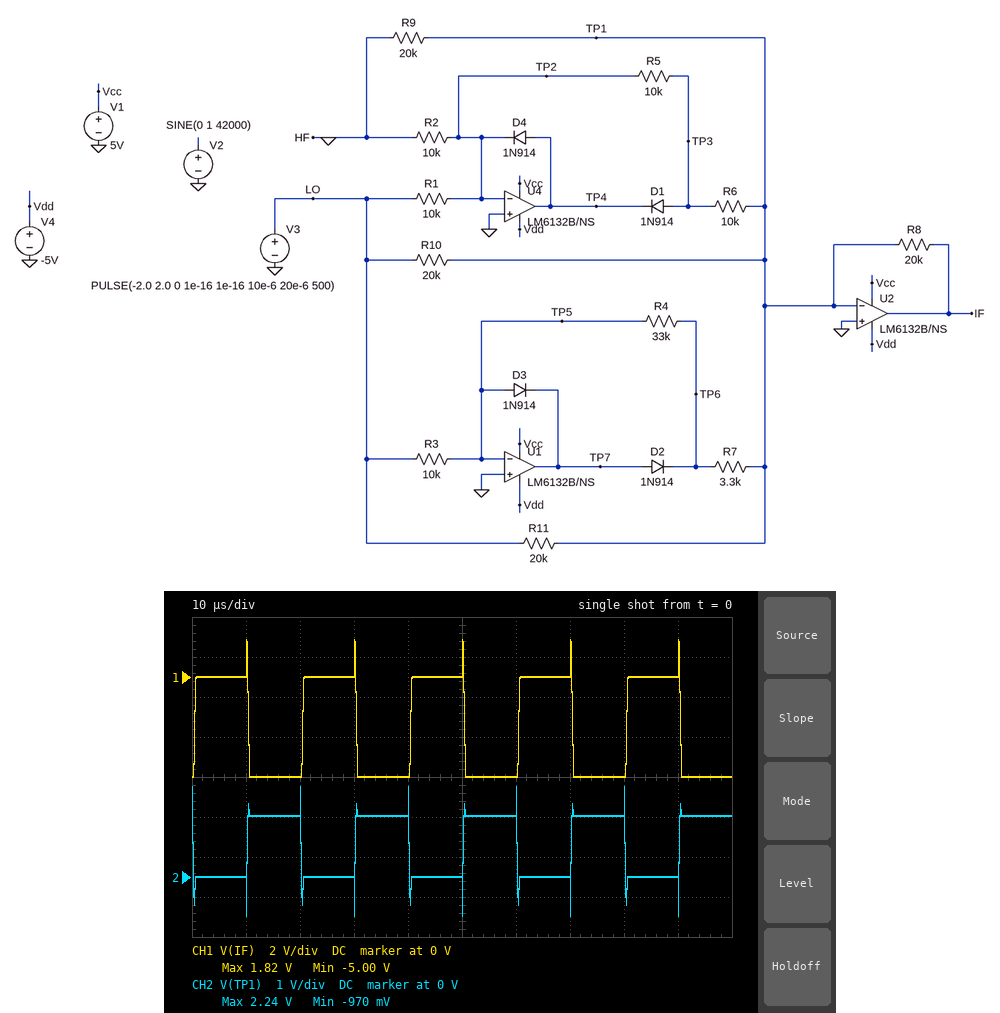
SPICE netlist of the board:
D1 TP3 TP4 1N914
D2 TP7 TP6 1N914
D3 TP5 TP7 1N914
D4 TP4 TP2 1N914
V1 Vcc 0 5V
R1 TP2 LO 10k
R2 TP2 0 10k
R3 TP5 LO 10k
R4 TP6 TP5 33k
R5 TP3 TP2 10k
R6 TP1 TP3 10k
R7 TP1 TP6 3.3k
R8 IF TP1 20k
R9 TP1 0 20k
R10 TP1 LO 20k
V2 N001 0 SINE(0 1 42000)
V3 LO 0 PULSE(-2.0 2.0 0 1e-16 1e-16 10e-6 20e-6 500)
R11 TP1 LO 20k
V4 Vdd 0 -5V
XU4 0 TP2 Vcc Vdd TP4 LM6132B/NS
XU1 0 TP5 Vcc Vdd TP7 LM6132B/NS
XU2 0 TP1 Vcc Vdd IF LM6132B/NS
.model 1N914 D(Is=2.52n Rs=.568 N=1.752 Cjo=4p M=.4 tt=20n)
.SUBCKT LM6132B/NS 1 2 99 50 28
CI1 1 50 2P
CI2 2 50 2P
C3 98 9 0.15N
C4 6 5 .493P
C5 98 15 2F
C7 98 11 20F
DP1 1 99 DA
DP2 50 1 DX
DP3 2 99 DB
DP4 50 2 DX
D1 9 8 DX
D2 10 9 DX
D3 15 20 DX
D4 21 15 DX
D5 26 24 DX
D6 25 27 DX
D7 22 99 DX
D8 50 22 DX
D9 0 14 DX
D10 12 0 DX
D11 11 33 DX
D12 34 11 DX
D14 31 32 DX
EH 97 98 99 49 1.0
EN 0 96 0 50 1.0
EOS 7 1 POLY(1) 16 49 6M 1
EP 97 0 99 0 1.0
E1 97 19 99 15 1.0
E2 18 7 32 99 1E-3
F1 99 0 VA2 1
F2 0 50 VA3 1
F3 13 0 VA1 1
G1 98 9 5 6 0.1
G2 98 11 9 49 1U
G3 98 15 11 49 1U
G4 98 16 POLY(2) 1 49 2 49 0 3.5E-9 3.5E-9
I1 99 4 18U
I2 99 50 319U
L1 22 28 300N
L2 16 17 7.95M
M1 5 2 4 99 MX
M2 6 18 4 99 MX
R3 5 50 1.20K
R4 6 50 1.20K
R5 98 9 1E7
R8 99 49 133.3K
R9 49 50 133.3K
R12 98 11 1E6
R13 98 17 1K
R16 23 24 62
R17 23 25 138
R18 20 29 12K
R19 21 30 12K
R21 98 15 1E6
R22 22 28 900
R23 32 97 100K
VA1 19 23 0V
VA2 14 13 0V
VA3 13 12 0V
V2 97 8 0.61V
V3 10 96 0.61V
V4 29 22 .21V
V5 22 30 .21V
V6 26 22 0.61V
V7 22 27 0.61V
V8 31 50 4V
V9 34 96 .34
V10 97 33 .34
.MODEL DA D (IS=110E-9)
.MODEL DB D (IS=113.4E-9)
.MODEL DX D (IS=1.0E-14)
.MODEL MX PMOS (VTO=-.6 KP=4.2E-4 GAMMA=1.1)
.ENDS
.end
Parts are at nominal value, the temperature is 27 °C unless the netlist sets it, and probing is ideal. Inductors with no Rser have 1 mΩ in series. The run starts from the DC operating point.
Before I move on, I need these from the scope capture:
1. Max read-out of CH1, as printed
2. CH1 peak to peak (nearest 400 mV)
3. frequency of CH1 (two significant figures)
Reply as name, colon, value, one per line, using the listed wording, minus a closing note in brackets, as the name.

Max read-out of CH1, as printed: 1.82 V
CH1 peak to peak: 6.8 V
frequency of CH1: 50 kHz
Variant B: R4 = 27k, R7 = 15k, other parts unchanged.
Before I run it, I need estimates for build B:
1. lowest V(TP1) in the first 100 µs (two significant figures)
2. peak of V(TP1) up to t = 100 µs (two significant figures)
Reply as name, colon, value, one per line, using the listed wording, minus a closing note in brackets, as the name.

lowest V(TP1) in the first 100 µs: -1.1 V
peak of V(TP1) up to t = 100 µs: 1.2 V
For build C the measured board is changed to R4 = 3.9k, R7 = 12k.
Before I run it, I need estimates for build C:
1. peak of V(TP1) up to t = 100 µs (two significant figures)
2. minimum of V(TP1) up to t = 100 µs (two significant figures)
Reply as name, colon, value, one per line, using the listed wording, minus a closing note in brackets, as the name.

peak of V(TP1) up to t = 100 µs: 1.1 V
minimum of V(TP1) up to t = 100 µs: -1.1 V
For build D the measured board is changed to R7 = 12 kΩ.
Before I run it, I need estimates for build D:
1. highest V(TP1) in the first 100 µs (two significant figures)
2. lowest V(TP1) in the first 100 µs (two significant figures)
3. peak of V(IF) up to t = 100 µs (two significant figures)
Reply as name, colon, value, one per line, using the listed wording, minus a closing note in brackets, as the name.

highest V(TP1) in the first 100 µs: 1.1 V
lowest V(TP1) in the first 100 µs: -1.1 V
peak of V(IF) up to t = 100 µs: 2.4 V
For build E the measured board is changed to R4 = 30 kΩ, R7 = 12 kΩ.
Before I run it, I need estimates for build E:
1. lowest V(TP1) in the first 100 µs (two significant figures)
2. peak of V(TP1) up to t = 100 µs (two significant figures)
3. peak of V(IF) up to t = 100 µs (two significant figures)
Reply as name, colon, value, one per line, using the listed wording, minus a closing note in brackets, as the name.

lowest V(TP1) in the first 100 µs: -1.1 V
peak of V(TP1) up to t = 100 µs: 1.1 V
peak of V(IF) up to t = 100 µs: 2.4 V
